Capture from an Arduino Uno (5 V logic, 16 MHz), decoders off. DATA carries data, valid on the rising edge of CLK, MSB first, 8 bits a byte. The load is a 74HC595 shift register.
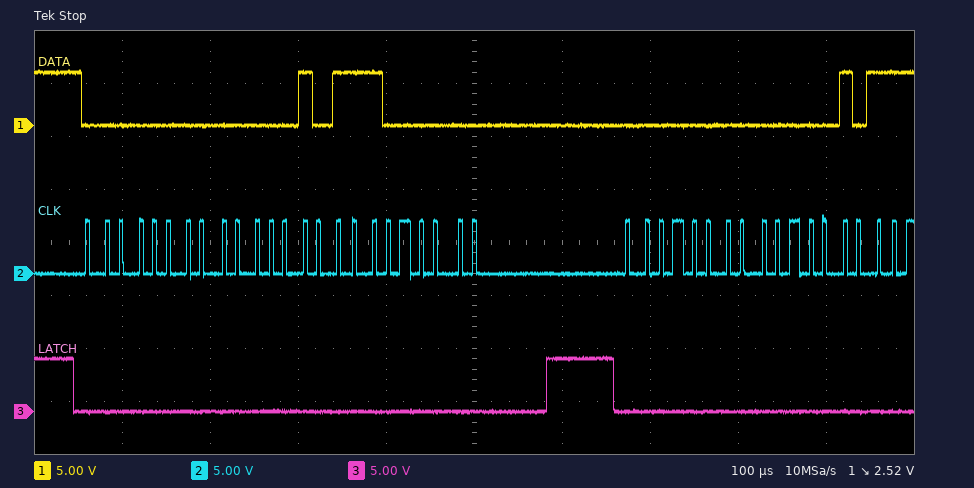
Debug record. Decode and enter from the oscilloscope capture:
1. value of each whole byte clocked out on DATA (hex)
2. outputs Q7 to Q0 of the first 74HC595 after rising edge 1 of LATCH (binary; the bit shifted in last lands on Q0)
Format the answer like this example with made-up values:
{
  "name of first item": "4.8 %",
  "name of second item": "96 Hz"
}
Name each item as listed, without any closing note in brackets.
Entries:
{
  "value of each whole byte clocked out on DATA": "0x00 0x05 0xC0 0x00 0x05",
  "outputs Q7 to Q0 of the first 74HC595 after rising edge 1 of LATCH": "11000000"
}
